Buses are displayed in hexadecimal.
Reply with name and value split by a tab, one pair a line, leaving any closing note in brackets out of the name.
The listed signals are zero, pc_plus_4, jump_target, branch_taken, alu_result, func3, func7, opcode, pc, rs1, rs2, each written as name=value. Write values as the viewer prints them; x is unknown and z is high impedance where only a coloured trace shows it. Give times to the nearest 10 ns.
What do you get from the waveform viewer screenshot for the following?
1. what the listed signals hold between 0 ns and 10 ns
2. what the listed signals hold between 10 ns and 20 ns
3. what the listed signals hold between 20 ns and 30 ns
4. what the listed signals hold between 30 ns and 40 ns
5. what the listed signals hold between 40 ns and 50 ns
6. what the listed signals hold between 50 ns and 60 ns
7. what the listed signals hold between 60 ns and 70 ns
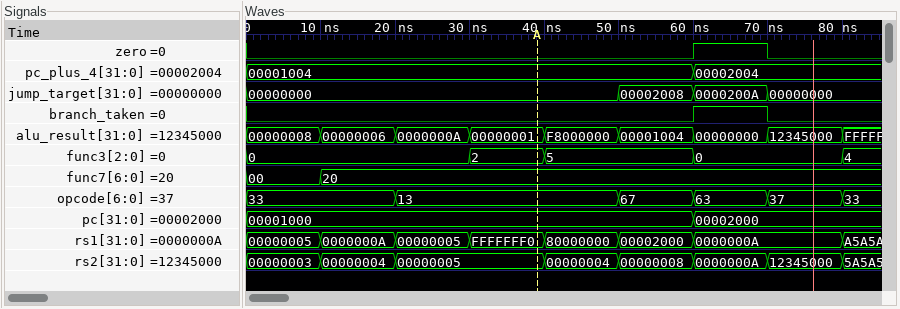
what the listed signals hold between 0 ns and 10 ns	zero=0, pc_plus_4=00001004, jump_target=00000000, branch_taken=0, alu_result=00000008, func3=0, func7=00, opcode=33, pc=00001000, rs1=00000005, rs2=00000003
what the listed signals hold between 10 ns and 20 ns	zero=0, pc_plus_4=00001004, jump_target=00000000, branch_taken=0, alu_result=00000006, func3=0, func7=20, opcode=33, pc=00001000, rs1=0000000A, rs2=00000004
what the listed signals hold between 20 ns and 30 ns	zero=0, pc_plus_4=00001004, jump_target=00000000, branch_taken=0, alu_result=0000000A, func3=0, func7=20, opcode=13, pc=00001000, rs1=00000005, rs2=00000005
what the listed signals hold between 30 ns and 40 ns	zero=0, pc_plus_4=00001004, jump_target=00000000, branch_taken=0, alu_result=00000001, func3=2, func7=20, opcode=13, pc=00001000, rs1=FFFFFFF0, rs2=00000005
what the listed signals hold between 40 ns and 50 ns	zero=0, pc_plus_4=00001004, jump_target=00000000, branch_taken=0, alu_result=F8000000, func3=5, func7=20, opcode=13, pc=00001000, rs1=80000000, rs2=00000004
what the listed signals hold between 50 ns and 60 ns	zero=0, pc_plus_4=00001004, jump_target=00002008, branch_taken=0, alu_result=00001004, func3=5, func7=20, opcode=67, pc=00001000, rs1=00002000, rs2=00000008
what the listed signals hold between 60 ns and 70 ns	zero=1, pc_plus_4=00002004, jump_target=0000200A, branch_taken=1, alu_result=00000000, func3=0, func7=20, opcode=63, pc=00002000, rs1=0000000A, rs2=0000000A
